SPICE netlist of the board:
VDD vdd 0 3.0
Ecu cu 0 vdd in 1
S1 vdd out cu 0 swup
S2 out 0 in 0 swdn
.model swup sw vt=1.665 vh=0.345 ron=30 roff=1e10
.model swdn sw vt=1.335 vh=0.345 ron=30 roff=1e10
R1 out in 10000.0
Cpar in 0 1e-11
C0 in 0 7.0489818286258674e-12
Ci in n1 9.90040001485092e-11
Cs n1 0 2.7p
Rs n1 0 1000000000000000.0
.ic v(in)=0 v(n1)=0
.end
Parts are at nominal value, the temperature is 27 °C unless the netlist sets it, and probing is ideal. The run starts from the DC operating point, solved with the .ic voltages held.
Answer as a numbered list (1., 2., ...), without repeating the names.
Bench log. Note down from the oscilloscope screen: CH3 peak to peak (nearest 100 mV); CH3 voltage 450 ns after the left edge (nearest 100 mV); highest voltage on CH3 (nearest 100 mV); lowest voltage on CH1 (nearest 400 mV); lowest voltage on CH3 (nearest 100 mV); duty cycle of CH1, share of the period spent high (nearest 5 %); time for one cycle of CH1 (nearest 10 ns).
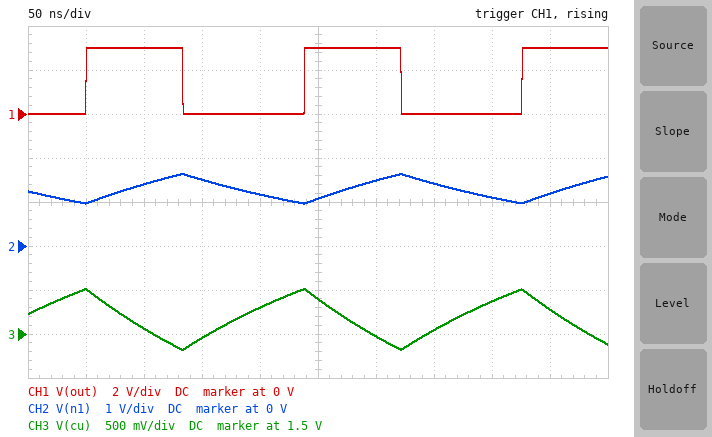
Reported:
1. 700 mV
2. 1.8 V
3. 2.0 V
4. 0 V
5. 1.3 V
6. 45 %
7. 190 ns
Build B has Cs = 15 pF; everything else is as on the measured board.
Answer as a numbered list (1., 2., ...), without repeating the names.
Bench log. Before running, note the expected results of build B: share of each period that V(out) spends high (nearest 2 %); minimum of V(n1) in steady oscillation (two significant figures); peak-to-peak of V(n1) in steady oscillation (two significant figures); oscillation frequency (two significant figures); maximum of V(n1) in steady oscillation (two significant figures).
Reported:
1. 44 %
2. 860 mV
3. 600 mV
4. 3.5 MHz
5. 1.5 V
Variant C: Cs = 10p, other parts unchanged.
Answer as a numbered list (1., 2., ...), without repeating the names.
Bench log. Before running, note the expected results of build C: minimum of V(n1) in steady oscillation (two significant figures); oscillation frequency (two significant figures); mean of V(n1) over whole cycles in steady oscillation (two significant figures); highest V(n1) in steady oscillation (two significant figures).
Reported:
1. 900 mV
2. 4.0 MHz
3. 1.2 V
4. 1.5 V
